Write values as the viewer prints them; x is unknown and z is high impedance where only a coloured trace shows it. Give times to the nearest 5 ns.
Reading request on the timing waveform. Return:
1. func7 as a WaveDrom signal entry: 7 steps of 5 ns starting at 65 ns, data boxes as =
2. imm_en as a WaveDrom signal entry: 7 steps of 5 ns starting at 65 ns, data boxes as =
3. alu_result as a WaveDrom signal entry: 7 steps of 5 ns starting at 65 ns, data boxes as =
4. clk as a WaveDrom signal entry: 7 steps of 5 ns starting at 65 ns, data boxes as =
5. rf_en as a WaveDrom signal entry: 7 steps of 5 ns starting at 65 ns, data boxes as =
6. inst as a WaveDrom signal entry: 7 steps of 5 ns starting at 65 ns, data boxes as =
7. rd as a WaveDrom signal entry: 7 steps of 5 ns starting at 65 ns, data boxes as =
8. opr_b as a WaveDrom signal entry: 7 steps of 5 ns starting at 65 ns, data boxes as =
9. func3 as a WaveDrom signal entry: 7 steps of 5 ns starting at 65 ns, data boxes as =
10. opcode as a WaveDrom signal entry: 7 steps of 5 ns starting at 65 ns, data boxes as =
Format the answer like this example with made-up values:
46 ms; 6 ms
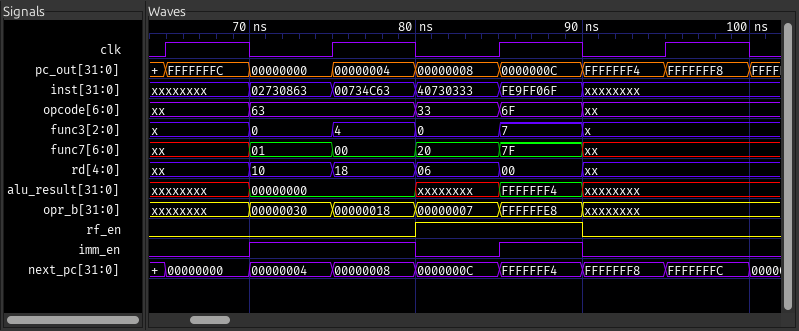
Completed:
{name: 'func7', wave: 'x====x.', data: '01 00 20 7F'}; {name: 'imm_en', wave: '01.010.'}; {name: 'alu_result', wave: 'x=.x=x.', data: '00000000 FFFFFFF4'}; {name: 'clk', wave: '1010101'}; {name: 'rf_en', wave: '0..1.0.'}; {name: 'inst', wave: 'x====x.', data: '02730863 00734C63 40730333 FE9FF06F'}; {name: 'rd', wave: 'x====x.', data: '10 18 06 00'}; {name: 'opr_b', wave: 'x====x.', data: '00000030 00000018 00000007 FFFFFFE8'}; {name: 'func3', wave: 'x====x.', data: '0 4 0 7'}; {name: 'opcode', wave: 'x=.==x.', data: '63 33 6F'}
